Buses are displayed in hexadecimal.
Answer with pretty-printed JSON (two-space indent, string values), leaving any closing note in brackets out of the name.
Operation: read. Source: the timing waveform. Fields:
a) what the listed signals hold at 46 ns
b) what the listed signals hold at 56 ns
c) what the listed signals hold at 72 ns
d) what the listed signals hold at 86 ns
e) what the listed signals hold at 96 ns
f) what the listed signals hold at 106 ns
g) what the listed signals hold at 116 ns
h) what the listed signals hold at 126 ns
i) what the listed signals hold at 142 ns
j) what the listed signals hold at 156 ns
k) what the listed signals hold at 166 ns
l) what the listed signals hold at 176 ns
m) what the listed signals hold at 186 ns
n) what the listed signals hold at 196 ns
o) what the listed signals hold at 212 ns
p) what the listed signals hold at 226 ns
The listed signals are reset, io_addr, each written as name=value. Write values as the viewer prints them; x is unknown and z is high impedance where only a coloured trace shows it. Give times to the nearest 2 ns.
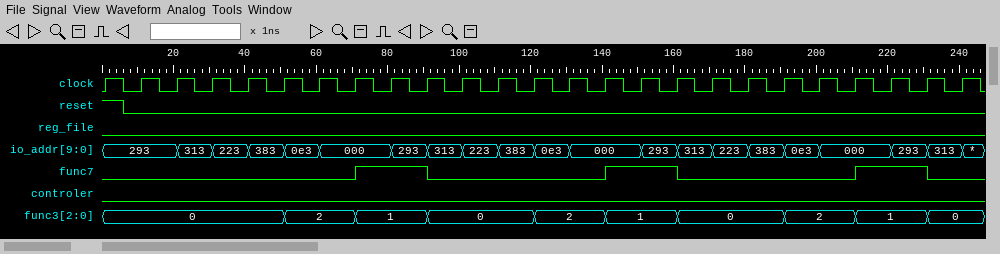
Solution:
{
  "what the listed signals hold at 46 ns": "reset=0, io_addr=383",
  "what the listed signals hold at 56 ns": "reset=0, io_addr=0e3",
  "what the listed signals hold at 72 ns": "reset=0, io_addr=000",
  "what the listed signals hold at 86 ns": "reset=0, io_addr=293",
  "what the listed signals hold at 96 ns": "reset=0, io_addr=313",
  "what the listed signals hold at 106 ns": "reset=0, io_addr=223",
  "what the listed signals hold at 116 ns": "reset=0, io_addr=383",
  "what the listed signals hold at 126 ns": "reset=0, io_addr=0e3",
  "what the listed signals hold at 142 ns": "reset=0, io_addr=000",
  "what the listed signals hold at 156 ns": "reset=0, io_addr=293",
  "what the listed signals hold at 166 ns": "reset=0, io_addr=313",
  "what the listed signals hold at 176 ns": "reset=0, io_addr=223",
  "what the listed signals hold at 186 ns": "reset=0, io_addr=383",
  "what the listed signals hold at 196 ns": "reset=0, io_addr=0e3",
  "what the listed signals hold at 212 ns": "reset=0, io_addr=000",
  "what the listed signals hold at 226 ns": "reset=0, io_addr=293"
}
